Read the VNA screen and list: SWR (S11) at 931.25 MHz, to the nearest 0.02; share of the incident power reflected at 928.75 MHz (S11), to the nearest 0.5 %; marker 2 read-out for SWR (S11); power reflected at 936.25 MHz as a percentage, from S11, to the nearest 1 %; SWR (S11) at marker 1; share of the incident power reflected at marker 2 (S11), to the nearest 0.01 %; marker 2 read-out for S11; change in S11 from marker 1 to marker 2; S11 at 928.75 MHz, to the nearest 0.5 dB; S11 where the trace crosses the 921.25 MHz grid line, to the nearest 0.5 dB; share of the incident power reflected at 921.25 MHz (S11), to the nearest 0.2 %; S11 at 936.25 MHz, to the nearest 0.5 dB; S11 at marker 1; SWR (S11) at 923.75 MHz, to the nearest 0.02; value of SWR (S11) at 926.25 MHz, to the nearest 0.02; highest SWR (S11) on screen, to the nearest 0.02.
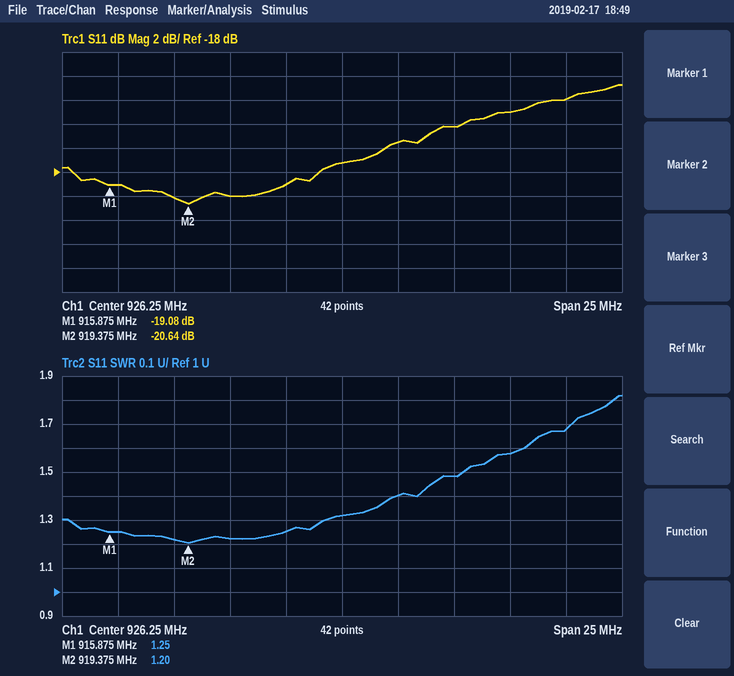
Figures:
1.48
3.0 %
1.20
6 %
1.25
0.86 %
-20.64 dB
-1.56 dB
-15.5 dB
-20.0 dB
1.0 %
-12.0 dB
-19.08 dB
1.26
1.32
1.82
